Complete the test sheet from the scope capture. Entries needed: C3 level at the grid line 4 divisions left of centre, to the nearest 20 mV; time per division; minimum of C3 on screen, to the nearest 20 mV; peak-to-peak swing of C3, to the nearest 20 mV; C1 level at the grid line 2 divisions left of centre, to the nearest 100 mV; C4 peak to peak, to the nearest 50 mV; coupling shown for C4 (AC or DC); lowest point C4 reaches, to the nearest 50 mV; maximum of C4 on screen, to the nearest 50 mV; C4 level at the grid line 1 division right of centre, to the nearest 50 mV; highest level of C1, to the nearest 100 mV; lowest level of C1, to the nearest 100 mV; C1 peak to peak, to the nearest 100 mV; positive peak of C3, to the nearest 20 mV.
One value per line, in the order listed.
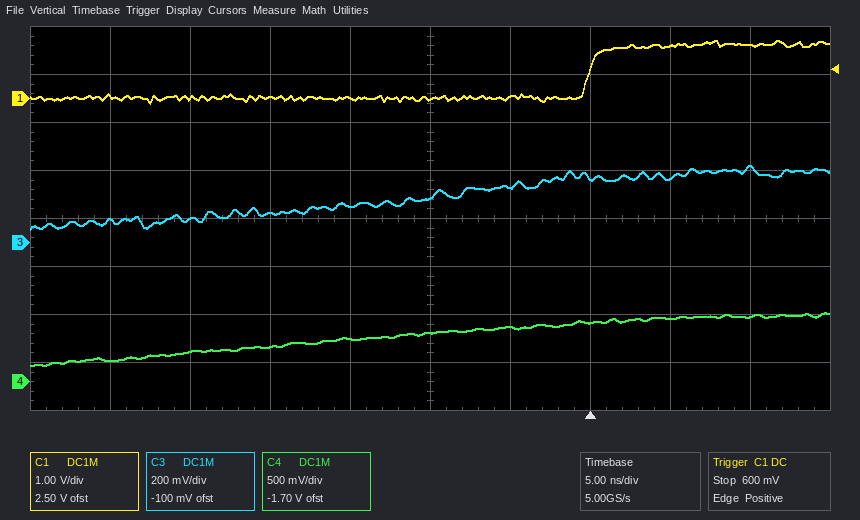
100 mV
5 ns
60 mV
260 mV
0.0 V
550 mV
DC
150 mV
700 mV
550 mV
1.2 V
-100 mV
1.3 V
320 mV
